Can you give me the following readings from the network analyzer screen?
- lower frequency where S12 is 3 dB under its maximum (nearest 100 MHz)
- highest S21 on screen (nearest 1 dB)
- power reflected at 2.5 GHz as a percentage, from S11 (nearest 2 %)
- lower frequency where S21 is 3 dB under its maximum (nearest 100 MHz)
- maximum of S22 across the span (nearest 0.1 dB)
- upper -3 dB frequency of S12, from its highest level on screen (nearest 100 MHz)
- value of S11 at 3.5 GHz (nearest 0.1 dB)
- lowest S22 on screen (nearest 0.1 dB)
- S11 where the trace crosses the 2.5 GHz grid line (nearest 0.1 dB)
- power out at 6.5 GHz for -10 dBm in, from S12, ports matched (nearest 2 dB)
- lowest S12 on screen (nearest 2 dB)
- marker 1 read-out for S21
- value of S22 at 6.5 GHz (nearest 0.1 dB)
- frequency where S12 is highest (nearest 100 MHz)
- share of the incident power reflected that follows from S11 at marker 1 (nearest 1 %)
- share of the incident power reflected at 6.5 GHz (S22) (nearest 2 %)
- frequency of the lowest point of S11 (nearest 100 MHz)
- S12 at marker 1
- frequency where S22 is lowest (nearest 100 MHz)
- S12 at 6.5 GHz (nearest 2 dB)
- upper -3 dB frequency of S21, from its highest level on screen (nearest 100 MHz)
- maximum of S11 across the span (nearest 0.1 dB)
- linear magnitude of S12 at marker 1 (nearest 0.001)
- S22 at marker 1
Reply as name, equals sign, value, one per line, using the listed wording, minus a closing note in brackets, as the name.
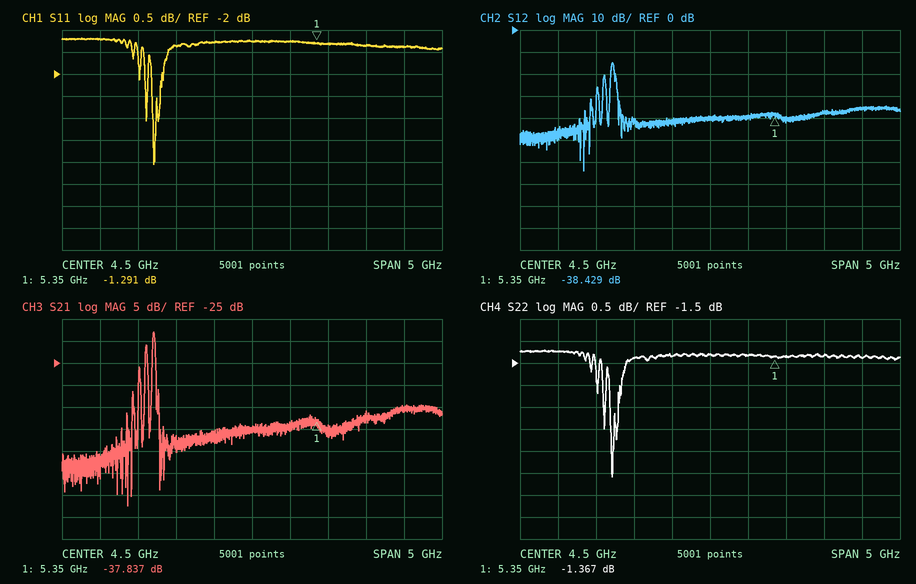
lower frequency where S12 is 3 dB under its maximum = 3.2 GHz
highest S21 on screen = -18 dB
power reflected at 2.5 GHz as a percentage, from S11 = 76 %
lower frequency where S21 is 3 dB under its maximum = 3.2 GHz
maximum of S22 across the span = -1.2 dB
upper -3 dB frequency of S12, from its highest level on screen = 3.2 GHz
value of S11 at 3.5 GHz = -1.4 dB
lowest S22 on screen = -4.1 dB
S11 where the trace crosses the 2.5 GHz grid line = -1.2 dB
power out at 6.5 GHz for -10 dBm in, from S12, ports matched = -46 dBm
lowest S12 on screen = -64 dB
marker 1 read-out for S21 = -37.837 dB
value of S22 at 6.5 GHz = -1.4 dB
frequency where S12 is highest = 3.2 GHz
share of the incident power reflected that follows from S11 at marker 1 = 74 %
share of the incident power reflected at 6.5 GHz (S22) = 72 %
frequency of the lowest point of S11 = 3.2 GHz
S12 at marker 1 = -38.429 dB
frequency where S22 is lowest = 3.2 GHz
S12 at 6.5 GHz = -36 dB
upper -3 dB frequency of S21, from its highest level on screen = 3.2 GHz
maximum of S11 across the span = -1.2 dB
linear magnitude of S12 at marker 1 = 0.012
S22 at marker 1 = -1.367 dB
